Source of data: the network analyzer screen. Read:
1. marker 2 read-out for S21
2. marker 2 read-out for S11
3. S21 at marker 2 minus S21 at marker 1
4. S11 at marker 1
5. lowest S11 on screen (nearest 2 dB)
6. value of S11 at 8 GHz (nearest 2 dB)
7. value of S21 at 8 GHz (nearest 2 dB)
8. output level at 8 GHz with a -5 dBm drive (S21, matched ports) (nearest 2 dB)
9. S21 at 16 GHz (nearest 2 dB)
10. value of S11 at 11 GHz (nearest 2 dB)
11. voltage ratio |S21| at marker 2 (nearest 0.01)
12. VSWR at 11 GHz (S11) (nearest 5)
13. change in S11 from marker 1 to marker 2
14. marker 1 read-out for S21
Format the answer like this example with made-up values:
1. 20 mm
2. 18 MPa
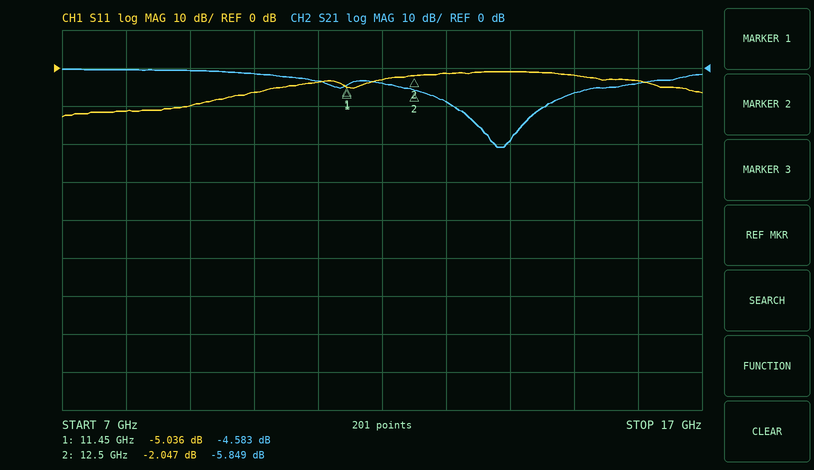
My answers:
1. -5.849 dB
2. -2.047 dB
3. -1.266 dB
4. -5.036 dB
5. -12 dB
6. -12 dB
7. 0 dB
8. -6 dBm
9. -4 dB
10. -4 dB
11. 0.51
12. 5
13. 2.989 dB
14. -4.583 dB
